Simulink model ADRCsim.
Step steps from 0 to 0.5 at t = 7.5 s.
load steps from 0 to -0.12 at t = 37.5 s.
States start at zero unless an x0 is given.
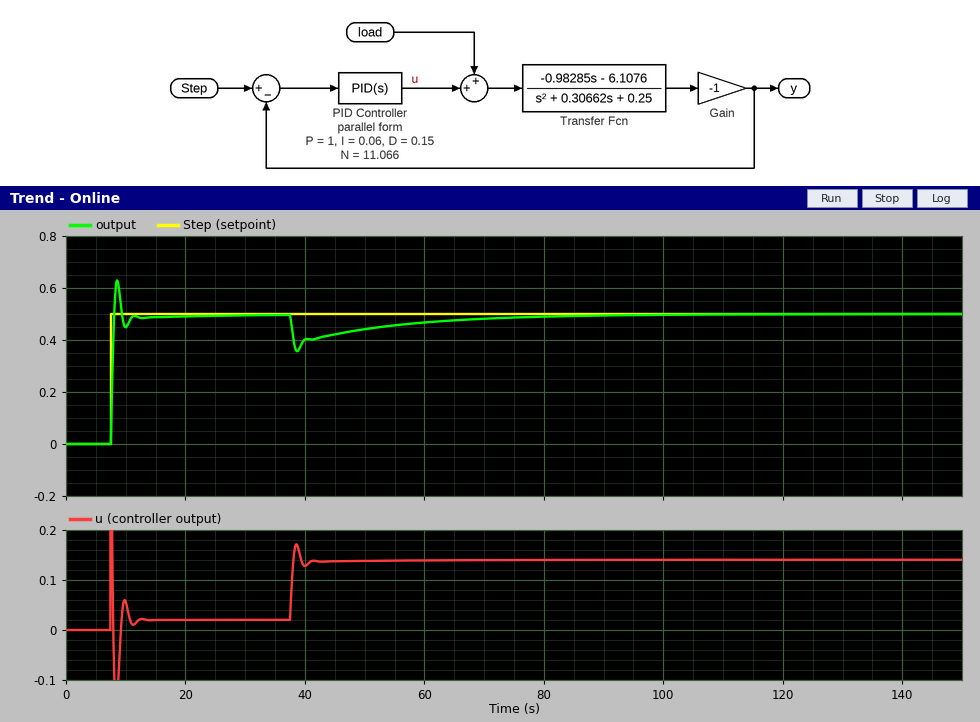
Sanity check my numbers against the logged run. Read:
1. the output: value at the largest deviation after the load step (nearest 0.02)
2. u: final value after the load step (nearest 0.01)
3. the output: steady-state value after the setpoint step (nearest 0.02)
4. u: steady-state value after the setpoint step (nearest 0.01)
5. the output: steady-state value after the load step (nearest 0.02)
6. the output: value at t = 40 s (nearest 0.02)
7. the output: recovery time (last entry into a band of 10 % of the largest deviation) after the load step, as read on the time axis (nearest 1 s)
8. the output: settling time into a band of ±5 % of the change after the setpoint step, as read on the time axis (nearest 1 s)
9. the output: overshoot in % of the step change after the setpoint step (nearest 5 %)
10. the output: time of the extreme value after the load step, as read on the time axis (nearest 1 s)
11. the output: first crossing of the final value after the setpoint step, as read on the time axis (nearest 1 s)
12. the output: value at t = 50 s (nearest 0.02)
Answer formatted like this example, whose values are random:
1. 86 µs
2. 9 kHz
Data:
1. 0.36
2. 0.14
3. 0.50
4. 0.02
5. 0.50
6. 0.40
7. 75 s
8. 11 s
9. 25 %
10. 39 s
11. 8 s
12. 0.44
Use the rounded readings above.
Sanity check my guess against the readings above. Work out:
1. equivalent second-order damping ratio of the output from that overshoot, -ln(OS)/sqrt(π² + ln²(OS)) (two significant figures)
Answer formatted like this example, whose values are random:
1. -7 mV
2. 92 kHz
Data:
1. 0.40
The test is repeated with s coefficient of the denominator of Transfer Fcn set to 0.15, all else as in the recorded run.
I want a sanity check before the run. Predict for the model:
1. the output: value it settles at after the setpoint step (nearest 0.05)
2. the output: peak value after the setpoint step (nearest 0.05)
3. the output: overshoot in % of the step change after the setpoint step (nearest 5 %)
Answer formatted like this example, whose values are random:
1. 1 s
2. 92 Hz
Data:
1. 0.50
2. 0.65
3. 30 %
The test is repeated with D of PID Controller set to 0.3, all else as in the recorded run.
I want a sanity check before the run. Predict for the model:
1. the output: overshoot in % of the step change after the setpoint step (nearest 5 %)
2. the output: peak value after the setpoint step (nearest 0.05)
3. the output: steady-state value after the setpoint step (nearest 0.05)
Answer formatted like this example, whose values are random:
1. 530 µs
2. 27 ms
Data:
1. 15 %
2. 0.60
3. 0.50
